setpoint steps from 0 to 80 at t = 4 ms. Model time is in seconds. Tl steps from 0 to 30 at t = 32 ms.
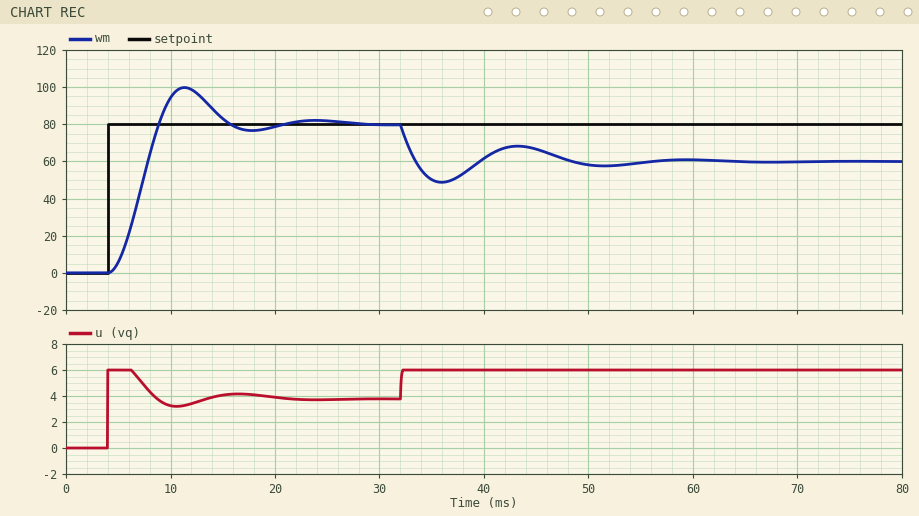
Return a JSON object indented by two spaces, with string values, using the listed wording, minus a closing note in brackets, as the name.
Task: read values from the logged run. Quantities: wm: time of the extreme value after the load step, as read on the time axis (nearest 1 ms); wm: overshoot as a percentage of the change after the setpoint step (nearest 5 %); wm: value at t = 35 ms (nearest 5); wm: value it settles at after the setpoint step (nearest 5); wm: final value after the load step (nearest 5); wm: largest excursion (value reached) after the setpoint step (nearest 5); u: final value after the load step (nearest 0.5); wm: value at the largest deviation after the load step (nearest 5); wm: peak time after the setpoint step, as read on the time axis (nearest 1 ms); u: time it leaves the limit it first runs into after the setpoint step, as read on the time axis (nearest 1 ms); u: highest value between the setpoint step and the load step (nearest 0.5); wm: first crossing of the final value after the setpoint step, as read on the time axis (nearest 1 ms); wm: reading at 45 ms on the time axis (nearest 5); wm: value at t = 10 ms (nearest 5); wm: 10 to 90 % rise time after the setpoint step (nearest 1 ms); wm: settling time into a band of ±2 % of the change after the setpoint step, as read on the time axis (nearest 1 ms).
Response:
{
  "wm: time of the extreme value after the load step, as read on the time axis": "36 ms",
  "wm: overshoot as a percentage of the change after the setpoint step": "25 %",
  "wm: value at t = 35 ms": "50",
  "wm: value it settles at after the setpoint step": "80",
  "wm: final value after the load step": "60",
  "wm: largest excursion (value reached) after the setpoint step": "100",
  "u: final value after the load step": "6.0",
  "wm: value at the largest deviation after the load step": "50",
  "wm: peak time after the setpoint step, as read on the time axis": "11 ms",
  "u: time it leaves the limit it first runs into after the setpoint step, as read on the time axis": "6 ms",
  "u: highest value between the setpoint step and the load step": "6.0",
  "wm: first crossing of the final value after the setpoint step, as read on the time axis": "9 ms",
  "wm: reading at 45 ms on the time axis": "65",
  "wm: value at t = 10 ms": "95",
  "wm: 10 to 90 % rise time after the setpoint step": "3 ms",
  "wm: settling time into a band of ±2 % of the change after the setpoint step, as read on the time axis": "26 ms"
}
